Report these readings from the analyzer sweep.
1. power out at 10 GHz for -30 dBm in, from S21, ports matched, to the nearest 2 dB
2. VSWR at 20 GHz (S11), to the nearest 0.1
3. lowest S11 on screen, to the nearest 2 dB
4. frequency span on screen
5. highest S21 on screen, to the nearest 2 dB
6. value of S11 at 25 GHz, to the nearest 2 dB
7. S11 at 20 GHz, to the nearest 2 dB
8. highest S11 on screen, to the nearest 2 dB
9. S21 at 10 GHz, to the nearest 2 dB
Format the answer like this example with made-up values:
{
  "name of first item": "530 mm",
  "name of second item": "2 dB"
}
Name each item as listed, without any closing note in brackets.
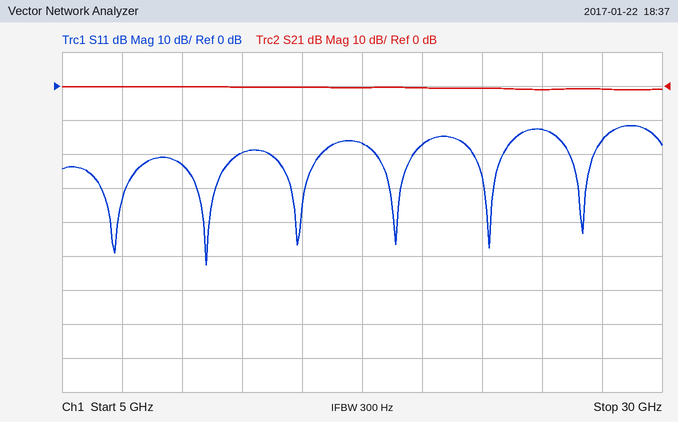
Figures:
{
  "power out at 10 GHz for -30 dBm in, from S21, ports matched, to the nearest 2 dB": "-30 dBm",
  "VSWR at 20 GHz (S11), to the nearest 0.1": "1.3",
  "lowest S11 on screen, to the nearest 2 dB": "-52 dB",
  "frequency span on screen": "25 GHz",
  "highest S21 on screen, to the nearest 2 dB": "0 dB",
  "value of S11 at 25 GHz, to the nearest 2 dB": "-12 dB",
  "S11 at 20 GHz, to the nearest 2 dB": "-18 dB",
  "highest S11 on screen, to the nearest 2 dB": "-12 dB",
  "S21 at 10 GHz, to the nearest 2 dB": "0 dB"
}
